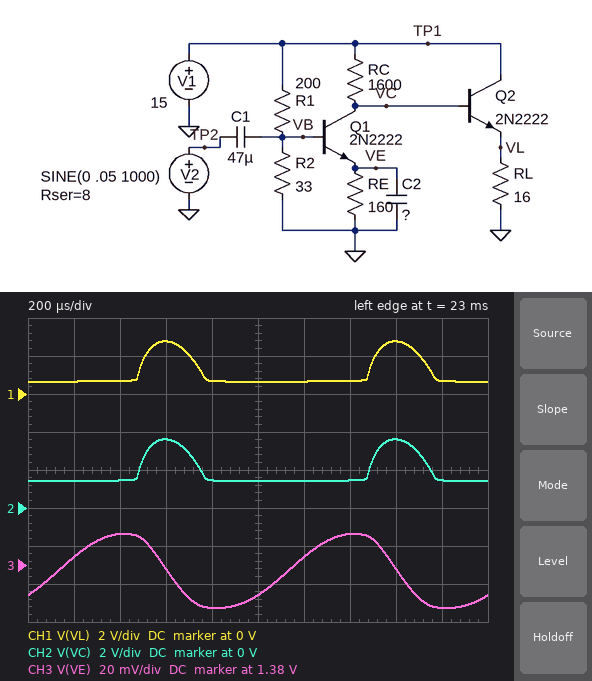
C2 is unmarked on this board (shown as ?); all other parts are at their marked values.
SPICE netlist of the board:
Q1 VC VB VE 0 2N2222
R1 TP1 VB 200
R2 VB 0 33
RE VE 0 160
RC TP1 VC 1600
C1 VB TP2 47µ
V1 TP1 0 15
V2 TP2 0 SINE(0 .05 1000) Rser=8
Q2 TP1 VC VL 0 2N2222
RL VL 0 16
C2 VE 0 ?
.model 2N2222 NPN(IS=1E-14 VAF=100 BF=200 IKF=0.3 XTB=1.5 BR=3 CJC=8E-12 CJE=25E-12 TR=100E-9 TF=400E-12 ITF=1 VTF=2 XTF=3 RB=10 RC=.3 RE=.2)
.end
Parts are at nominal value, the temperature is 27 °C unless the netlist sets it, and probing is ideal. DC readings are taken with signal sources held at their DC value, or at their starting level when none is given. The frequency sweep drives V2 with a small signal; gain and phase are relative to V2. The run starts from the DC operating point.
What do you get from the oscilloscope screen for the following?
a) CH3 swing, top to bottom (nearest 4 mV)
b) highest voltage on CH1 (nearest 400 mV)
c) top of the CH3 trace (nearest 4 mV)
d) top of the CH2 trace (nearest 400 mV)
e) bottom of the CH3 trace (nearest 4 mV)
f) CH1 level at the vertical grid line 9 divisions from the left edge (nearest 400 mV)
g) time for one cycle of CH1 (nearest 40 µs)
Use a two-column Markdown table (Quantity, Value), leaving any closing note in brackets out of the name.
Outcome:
| Quantity | Value |
|---|---|
| CH3 swing, top to bottom | 40 mV |
| highest voltage on CH1 | 2.8 V |
| top of the CH3 trace | 1.396 V |
| top of the CH2 trace | 3.6 V |
| bottom of the CH3 trace | 1.356 V |
| CH1 level at the vertical grid line 9 divisions from the left edge | 800 mV |
| time for one cycle of CH1 | 1.00 ms |
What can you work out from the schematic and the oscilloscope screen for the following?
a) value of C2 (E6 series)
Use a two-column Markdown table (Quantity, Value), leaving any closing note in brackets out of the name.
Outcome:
| Quantity | Value |
|---|---|
| value of C2 | 15 µF |
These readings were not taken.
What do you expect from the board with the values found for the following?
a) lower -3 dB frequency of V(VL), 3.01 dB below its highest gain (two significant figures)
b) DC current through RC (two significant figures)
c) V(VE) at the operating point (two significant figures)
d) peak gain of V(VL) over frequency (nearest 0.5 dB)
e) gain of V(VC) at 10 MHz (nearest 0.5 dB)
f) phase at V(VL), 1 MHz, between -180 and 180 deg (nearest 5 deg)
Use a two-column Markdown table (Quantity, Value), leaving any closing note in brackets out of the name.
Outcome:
| Quantity | Value |
|---|---|
| lower -3 dB frequency of V(VL), 3.01 dB below its highest gain | 550 Hz |
| DC current through RC | 8.5 mA |
| V(VE) at the operating point | 1.4 V |
| peak gain of V(VL) over frequency | 3.5 dB |
| gain of V(VC) at 10 MHz | -15.5 dB |
| phase at V(VL), 1 MHz, between -180 and 180 deg | 120 deg |
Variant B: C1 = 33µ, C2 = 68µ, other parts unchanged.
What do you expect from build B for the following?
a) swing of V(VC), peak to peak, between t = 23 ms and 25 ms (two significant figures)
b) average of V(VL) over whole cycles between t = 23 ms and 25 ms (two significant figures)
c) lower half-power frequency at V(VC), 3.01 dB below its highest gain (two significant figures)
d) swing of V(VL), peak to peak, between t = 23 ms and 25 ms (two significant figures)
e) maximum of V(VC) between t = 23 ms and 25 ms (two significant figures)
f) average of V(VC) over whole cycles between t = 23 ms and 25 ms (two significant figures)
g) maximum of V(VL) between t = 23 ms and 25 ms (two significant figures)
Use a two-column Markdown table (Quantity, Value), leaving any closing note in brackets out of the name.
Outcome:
| Quantity | Value |
|---|---|
| swing of V(VC), peak to peak, between t = 23 ms and 25 ms | 3.1 V |
| average of V(VL) over whole cycles between t = 23 ms and 25 ms | 1.3 V |
| lower half-power frequency at V(VC), 3.01 dB below its highest gain | 300 Hz |
| swing of V(VL), peak to peak, between t = 23 ms and 25 ms | 3.0 V |
| maximum of V(VC) between t = 23 ms and 25 ms | 4.5 V |
| average of V(VC) over whole cycles between t = 23 ms and 25 ms | 2.1 V |
| maximum of V(VL) between t = 23 ms and 25 ms | 3.6 V |
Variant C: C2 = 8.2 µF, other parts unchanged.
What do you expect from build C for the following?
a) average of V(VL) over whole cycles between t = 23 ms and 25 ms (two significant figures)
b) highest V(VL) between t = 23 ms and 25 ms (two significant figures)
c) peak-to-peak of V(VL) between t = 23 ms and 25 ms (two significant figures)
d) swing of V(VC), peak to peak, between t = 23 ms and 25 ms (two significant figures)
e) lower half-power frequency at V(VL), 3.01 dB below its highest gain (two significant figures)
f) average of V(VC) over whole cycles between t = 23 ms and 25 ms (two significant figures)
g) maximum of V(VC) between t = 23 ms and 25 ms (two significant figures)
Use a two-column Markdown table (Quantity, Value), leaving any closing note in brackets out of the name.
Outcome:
| Quantity | Value |
|---|---|
| average of V(VL) over whole cycles between t = 23 ms and 25 ms | 940 mV |
| highest V(VL) between t = 23 ms and 25 ms | 2.0 V |
| peak-to-peak of V(VL) between t = 23 ms and 25 ms | 1.3 V |
| swing of V(VC), peak to peak, between t = 23 ms and 25 ms | 1.4 V |
| lower half-power frequency at V(VL), 3.01 dB below its highest gain | 920 Hz |
| average of V(VC) over whole cycles between t = 23 ms and 25 ms | 1.7 V |
| maximum of V(VC) between t = 23 ms and 25 ms | 2.8 V |
